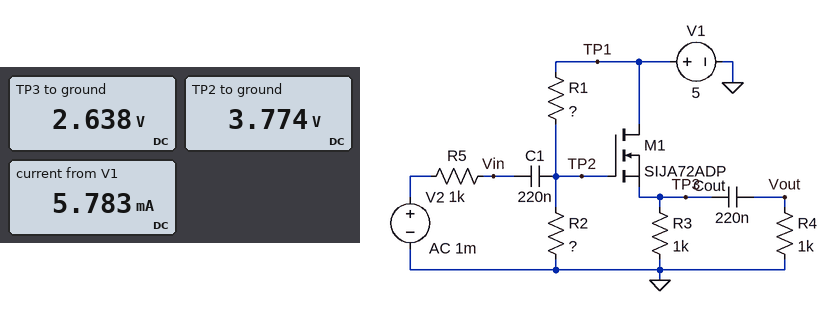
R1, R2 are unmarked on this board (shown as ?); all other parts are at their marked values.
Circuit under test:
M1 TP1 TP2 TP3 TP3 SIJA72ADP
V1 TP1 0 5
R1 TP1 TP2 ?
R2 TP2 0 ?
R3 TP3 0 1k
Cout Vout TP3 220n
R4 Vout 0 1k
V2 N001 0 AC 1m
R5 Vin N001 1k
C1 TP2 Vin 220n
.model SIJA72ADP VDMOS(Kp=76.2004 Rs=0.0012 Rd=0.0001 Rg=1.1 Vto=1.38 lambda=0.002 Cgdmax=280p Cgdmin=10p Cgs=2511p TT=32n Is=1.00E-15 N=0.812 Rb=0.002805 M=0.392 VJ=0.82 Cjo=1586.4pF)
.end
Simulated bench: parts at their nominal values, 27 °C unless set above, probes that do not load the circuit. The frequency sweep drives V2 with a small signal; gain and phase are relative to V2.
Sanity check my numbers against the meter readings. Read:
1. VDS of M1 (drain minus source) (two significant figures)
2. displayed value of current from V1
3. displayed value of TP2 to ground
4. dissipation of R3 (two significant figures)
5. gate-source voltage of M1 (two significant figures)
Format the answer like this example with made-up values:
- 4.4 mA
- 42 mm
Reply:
- 2.4 V
- 5.783 mA
- 3.774 V
- 7.0 mW
- 1.1 V
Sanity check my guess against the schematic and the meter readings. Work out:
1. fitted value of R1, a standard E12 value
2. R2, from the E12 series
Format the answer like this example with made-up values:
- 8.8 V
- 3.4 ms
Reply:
- 390 Ω
- 1.2 kΩ
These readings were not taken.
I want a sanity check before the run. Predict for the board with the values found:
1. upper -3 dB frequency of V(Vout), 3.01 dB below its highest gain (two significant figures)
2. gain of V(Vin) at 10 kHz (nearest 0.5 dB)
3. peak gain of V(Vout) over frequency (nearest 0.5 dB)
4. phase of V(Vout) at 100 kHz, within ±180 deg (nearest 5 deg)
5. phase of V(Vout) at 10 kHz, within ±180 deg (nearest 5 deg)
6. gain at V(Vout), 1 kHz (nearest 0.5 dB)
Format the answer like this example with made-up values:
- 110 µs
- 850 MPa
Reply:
- 1.8 MHz
- -12.5 dB
- -11.5 dB
- 0 deg
- 5 deg
- -16.0 dB
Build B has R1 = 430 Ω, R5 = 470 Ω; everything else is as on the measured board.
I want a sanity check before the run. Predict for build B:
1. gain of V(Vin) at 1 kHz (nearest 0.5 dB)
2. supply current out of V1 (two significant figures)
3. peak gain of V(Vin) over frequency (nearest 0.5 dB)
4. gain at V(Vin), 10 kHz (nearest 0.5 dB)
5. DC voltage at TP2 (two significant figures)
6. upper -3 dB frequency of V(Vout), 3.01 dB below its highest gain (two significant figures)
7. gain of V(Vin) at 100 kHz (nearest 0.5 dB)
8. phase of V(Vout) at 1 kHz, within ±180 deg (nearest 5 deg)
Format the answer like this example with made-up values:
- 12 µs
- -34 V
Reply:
- -2.5 dB
- 5.6 mA
- 0 dB
- -7.5 dB
- 3.7 V
- 2.0 MHz
- -8.0 dB
- 80 deg
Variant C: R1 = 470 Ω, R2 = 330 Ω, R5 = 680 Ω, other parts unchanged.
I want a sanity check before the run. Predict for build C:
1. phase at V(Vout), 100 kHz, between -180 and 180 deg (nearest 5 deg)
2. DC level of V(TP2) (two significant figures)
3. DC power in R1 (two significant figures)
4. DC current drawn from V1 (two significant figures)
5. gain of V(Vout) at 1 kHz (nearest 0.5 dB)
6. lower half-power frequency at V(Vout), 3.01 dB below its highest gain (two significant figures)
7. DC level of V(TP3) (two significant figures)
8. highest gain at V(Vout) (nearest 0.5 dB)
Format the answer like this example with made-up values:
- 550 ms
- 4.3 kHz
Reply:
- 0 deg
- 2.1 V
- 18 mW
- 7.2 mA
- -18.0 dB
- 1.2 kHz
- 980 mV
- -13.5 dB
